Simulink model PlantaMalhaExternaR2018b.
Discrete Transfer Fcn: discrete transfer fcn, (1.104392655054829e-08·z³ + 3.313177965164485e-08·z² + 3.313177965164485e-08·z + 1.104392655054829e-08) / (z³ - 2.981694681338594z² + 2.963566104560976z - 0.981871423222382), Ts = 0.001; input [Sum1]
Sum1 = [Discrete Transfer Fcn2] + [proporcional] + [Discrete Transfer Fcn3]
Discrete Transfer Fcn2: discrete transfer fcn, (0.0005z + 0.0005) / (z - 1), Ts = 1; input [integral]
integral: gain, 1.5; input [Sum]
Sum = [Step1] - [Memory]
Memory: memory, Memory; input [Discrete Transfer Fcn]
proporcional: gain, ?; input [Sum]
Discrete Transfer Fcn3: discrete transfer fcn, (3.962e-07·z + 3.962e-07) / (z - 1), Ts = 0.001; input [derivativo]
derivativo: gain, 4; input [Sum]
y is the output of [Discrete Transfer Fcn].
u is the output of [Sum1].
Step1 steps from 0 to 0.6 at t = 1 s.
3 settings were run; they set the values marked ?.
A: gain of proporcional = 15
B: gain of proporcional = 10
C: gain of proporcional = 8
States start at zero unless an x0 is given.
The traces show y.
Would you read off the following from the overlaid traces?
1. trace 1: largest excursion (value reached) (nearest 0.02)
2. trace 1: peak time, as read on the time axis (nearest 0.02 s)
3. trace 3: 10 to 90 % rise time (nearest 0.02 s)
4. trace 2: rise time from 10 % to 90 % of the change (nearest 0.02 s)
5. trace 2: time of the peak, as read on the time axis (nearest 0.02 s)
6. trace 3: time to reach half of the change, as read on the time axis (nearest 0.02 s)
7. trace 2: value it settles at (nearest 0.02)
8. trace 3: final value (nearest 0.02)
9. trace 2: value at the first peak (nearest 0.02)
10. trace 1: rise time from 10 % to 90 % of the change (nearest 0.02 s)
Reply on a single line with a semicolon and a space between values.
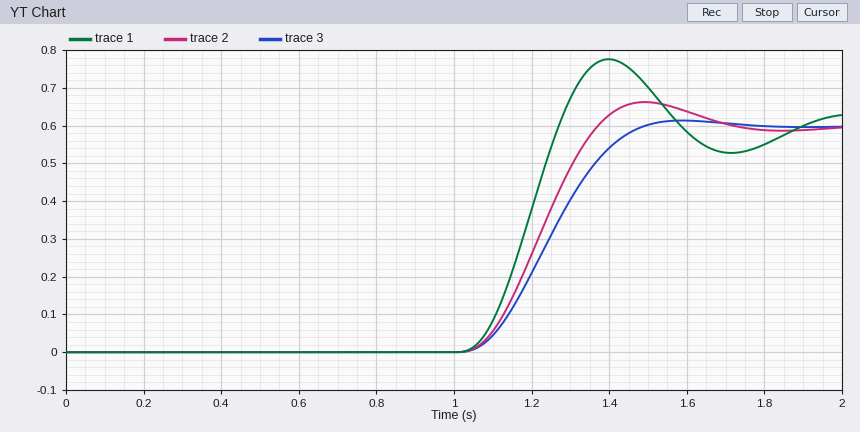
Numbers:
0.78; 1.40 s; 0.28 s; 0.22 s; 1.50 s; 1.24 s; 0.60; 0.60; 0.66; 0.16 s
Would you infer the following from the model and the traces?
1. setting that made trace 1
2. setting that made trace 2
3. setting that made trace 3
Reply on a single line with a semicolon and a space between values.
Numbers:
A; B; C
